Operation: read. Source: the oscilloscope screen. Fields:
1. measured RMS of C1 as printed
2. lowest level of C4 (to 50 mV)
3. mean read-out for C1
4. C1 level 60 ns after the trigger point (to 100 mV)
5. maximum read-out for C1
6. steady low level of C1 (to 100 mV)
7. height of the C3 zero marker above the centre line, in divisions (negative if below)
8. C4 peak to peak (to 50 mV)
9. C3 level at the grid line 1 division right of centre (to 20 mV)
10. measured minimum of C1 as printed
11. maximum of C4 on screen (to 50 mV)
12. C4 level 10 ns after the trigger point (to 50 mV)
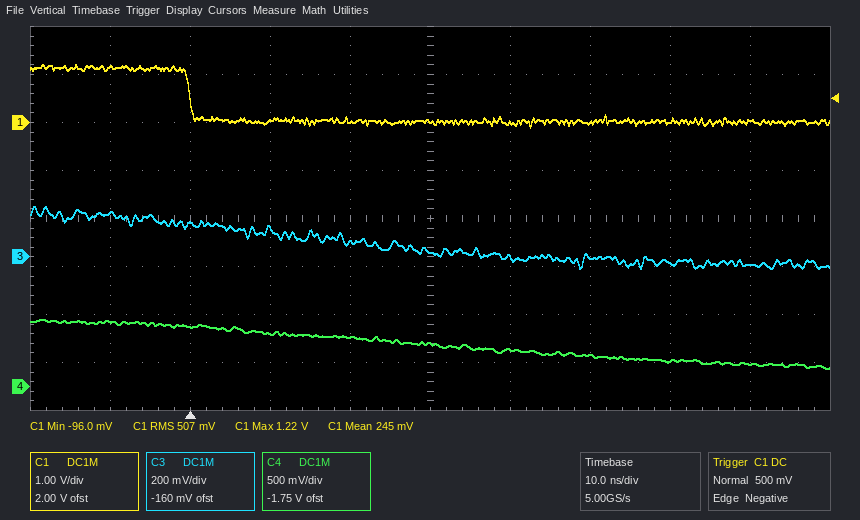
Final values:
507 mV
200 mV
245 mV
0.0 V
1.22 V
0.0 V
-0.8 div
500 mV
0 mV
-96.0 mV
700 mV
550 mV
